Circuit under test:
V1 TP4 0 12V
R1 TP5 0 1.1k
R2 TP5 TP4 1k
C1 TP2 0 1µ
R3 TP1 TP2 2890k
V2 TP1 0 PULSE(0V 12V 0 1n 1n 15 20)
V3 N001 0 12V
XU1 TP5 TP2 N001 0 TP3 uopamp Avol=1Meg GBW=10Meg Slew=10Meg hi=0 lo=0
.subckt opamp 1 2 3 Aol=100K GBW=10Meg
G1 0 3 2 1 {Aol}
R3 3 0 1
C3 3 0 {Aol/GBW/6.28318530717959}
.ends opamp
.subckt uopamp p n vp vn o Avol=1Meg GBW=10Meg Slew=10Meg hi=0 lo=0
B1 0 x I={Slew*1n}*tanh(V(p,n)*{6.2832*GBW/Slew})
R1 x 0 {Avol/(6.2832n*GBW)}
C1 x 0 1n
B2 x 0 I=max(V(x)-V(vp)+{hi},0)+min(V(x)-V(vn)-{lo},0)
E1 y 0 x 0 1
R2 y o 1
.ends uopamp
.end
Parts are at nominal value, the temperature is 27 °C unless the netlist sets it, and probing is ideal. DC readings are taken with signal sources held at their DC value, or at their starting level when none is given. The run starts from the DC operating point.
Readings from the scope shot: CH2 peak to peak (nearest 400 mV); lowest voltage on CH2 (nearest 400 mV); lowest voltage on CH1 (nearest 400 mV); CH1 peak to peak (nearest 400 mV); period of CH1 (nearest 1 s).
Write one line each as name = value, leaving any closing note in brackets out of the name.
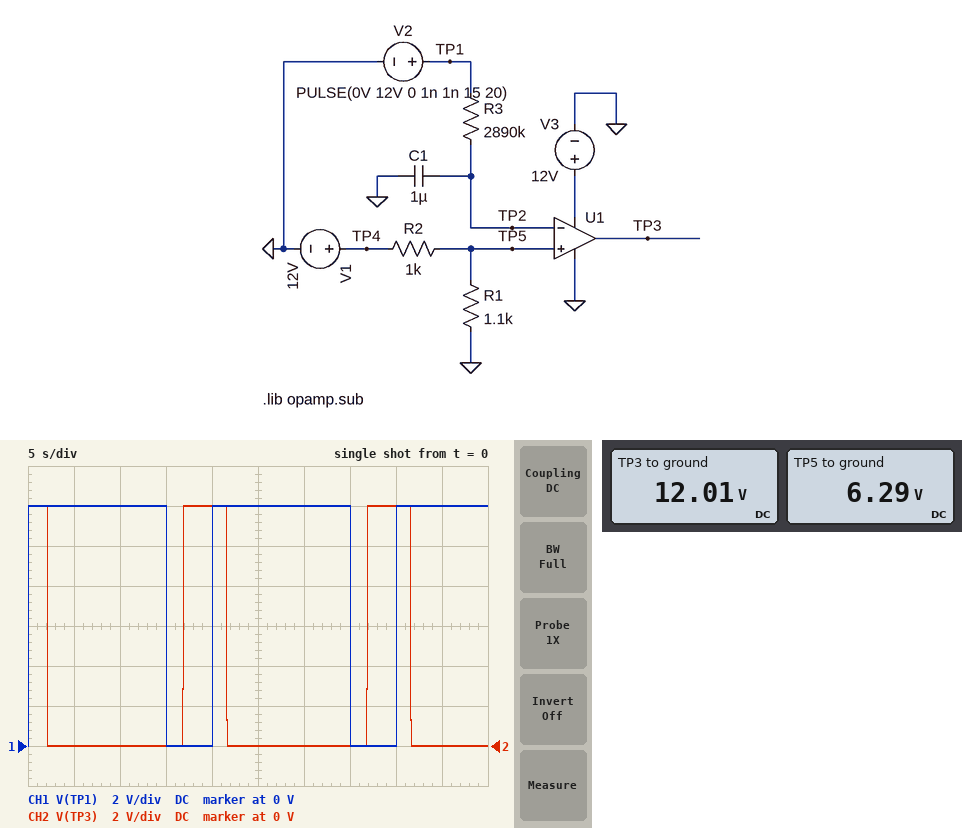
CH2 peak to peak = 12.0 V
lowest voltage on CH2 = 0 V
lowest voltage on CH1 = 0 V
CH1 peak to peak = 12.0 V
period of CH1 = 20 s
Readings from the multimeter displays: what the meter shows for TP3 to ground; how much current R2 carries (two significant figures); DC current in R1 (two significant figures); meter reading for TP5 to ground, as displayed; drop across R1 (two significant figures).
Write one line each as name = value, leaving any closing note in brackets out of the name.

what the meter shows for TP3 to ground = 12.01 V
how much current R2 carries = 5.7 mA
DC current in R1 = 5.7 mA
meter reading for TP5 to ground, as displayed = 6.29 V
drop across R1 = 6.3 V
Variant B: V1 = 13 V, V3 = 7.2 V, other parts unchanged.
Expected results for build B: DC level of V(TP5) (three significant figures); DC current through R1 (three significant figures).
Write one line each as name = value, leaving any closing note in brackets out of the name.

DC level of V(TP5) = 6.81 V
DC current through R1 = 6.19 mA
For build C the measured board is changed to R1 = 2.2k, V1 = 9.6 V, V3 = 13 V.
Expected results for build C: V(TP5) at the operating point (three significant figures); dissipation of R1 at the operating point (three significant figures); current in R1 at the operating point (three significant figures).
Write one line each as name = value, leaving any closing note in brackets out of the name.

V(TP5) at the operating point = 6.60 V
dissipation of R1 at the operating point = 19.8 mW
current in R1 at the operating point = 3.00 mA
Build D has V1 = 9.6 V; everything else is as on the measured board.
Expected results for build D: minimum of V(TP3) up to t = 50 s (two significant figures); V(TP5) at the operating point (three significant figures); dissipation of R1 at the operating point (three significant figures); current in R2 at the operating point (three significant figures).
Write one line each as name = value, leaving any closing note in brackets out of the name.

minimum of V(TP3) up to t = 50 s = -10 mV
V(TP5) at the operating point = 5.03 V
dissipation of R1 at the operating point = 23.0 mW
current in R2 at the operating point = 4.57 mA
